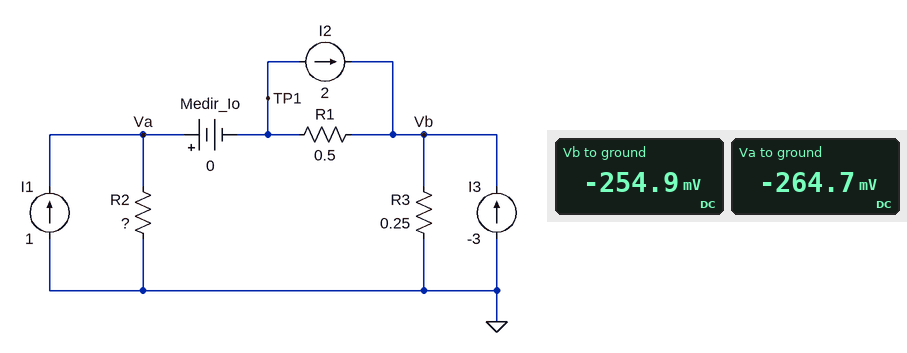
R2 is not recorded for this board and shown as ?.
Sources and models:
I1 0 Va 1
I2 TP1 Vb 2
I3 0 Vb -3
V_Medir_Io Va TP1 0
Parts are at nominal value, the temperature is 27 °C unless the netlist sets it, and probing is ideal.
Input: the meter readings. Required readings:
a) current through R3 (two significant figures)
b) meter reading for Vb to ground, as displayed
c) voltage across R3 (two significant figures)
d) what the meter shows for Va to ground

1.0 A
-254.9 mV
250 mV
-264.7 mV
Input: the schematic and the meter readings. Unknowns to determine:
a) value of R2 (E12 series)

0.27 Ω
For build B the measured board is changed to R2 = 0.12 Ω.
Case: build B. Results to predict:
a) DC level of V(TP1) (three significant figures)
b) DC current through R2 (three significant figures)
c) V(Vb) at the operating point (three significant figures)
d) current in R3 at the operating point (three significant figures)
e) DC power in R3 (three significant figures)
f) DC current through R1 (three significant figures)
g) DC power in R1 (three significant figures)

-138 mV
1.15 A
-213 mV
851 mA
181 mW
149 mA
11.2 mW
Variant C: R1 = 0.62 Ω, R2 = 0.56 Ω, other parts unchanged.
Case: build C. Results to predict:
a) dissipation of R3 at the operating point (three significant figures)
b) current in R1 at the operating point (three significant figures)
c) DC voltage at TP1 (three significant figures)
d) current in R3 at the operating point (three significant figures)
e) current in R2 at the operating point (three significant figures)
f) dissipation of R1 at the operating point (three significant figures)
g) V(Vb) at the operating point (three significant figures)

370 mW
217 mA
-439 mV
1.22 A
783 mA
29.1 mW
-304 mV
